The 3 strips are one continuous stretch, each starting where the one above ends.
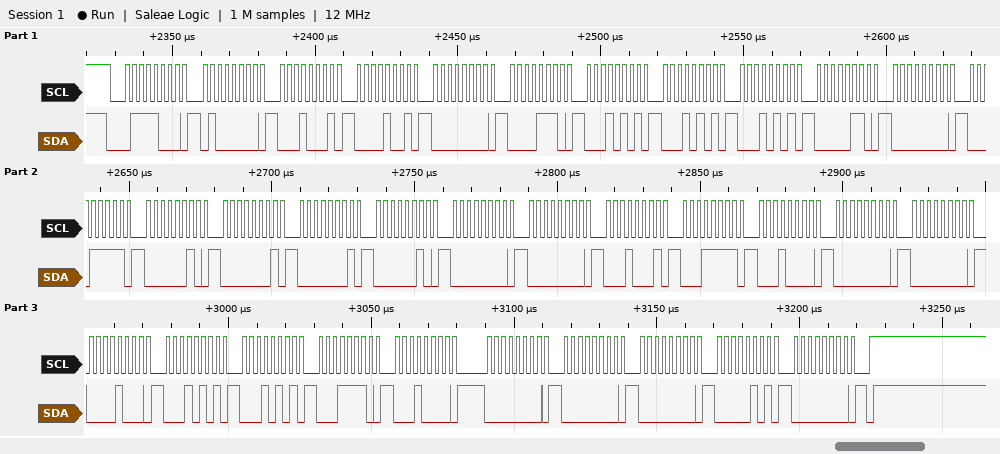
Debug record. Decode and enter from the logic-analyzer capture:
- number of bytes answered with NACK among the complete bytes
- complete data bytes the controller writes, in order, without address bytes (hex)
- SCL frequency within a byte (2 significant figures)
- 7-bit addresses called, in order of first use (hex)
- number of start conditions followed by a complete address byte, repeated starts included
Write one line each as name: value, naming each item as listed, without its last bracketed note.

number of bytes answered with NACK among the complete bytes: 0
complete data bytes the controller writes, in order, without address bytes: 40 11 09 00 0E 15 15 15 06 00 1F 02 01 01 02 00 00 11 1F 10 00 00 08 15 15 1E 10 00 00 00 05 00
SCL frequency within a byte: 400 kHz
7-bit addresses called, in order of first use: 0x3C
number of start conditions followed by a complete address byte, repeated starts included: 1
